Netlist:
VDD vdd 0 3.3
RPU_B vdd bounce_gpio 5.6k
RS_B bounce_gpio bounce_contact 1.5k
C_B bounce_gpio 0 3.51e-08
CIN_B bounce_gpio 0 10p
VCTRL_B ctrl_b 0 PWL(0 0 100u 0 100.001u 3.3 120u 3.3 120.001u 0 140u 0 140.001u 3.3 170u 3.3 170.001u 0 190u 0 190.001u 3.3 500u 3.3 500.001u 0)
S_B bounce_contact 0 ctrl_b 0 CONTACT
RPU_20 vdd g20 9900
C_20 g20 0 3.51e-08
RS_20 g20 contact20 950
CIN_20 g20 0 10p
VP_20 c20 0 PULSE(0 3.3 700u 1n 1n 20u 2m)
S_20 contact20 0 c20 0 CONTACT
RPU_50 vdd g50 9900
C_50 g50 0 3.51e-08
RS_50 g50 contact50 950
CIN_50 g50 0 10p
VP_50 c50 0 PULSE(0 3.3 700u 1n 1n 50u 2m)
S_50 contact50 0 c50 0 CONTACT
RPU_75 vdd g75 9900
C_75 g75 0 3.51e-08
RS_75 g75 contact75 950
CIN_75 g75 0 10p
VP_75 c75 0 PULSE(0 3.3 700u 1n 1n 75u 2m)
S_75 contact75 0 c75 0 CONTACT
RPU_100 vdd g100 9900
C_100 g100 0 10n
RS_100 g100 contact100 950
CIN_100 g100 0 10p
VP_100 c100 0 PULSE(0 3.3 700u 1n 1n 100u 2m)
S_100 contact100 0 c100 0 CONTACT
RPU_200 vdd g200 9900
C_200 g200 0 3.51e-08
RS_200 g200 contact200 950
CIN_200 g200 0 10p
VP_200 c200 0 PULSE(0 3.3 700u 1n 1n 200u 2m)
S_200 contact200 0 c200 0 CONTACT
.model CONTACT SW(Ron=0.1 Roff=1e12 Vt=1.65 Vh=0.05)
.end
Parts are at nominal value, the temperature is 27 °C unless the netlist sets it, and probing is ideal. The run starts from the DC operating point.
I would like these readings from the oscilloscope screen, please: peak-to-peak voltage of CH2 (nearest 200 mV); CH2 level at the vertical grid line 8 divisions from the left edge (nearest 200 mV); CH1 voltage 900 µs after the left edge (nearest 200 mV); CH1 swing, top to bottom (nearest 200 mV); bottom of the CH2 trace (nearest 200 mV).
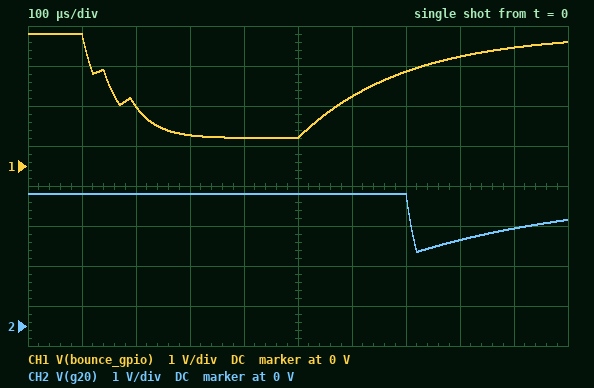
1.4 V
2.2 V
3.0 V
2.6 V
1.8 V
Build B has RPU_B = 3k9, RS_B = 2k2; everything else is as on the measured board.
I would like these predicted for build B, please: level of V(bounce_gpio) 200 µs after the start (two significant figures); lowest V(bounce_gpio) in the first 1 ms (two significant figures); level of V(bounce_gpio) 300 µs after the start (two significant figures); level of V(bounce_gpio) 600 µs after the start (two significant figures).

2.0 V
1.2 V
1.3 V
2.3 V
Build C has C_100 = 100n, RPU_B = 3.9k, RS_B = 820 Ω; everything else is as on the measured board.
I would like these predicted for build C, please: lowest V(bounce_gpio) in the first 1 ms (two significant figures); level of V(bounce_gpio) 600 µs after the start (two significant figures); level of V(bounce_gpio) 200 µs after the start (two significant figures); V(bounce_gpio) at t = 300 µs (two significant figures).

570 mV
2.0 V
1.0 V
580 mV
